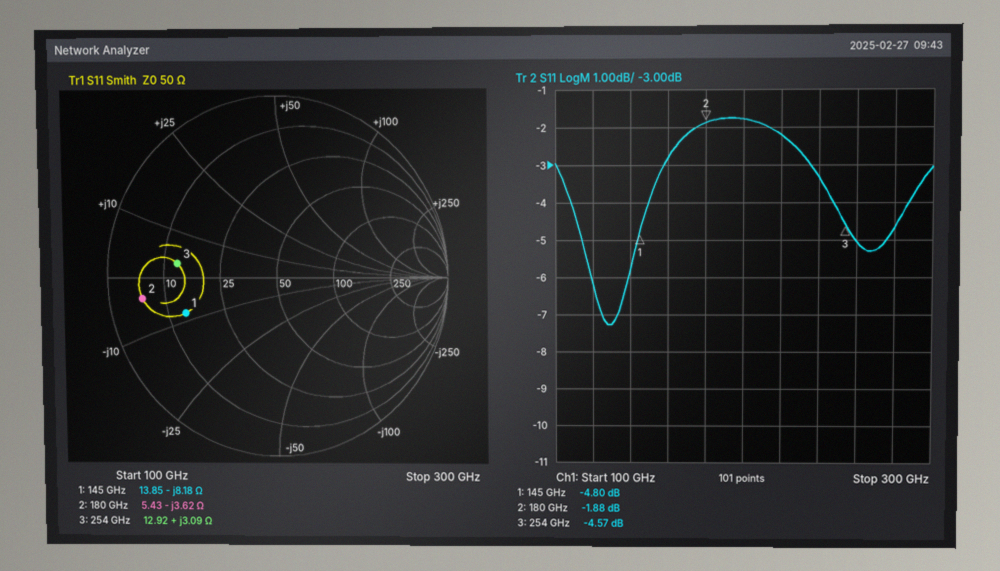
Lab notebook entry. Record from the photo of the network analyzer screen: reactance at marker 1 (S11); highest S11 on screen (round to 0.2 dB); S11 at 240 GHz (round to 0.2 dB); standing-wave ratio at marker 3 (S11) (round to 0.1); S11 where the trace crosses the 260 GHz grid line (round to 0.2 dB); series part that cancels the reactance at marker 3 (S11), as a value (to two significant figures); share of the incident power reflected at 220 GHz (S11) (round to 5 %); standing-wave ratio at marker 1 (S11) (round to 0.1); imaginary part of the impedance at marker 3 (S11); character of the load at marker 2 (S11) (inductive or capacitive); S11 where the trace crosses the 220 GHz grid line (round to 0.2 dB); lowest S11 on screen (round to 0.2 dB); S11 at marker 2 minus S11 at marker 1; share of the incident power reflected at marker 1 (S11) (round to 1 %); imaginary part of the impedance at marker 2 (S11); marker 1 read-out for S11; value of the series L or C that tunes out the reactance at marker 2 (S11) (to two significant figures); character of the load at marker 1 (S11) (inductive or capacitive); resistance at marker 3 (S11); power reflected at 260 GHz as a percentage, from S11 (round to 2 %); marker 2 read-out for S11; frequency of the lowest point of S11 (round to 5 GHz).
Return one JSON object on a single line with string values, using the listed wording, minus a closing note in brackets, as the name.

{"reactance at marker 1": "-8.18 Ω", "highest S11 on screen": "-1.8 dB", "S11 at 240 GHz": "-3.4 dB", "standing-wave ratio at marker 3 (S11)": "3.9", "S11 where the trace crosses the 260 GHz grid line": "-5.0 dB", "series part that cancels the reactance at marker 3 (S11), as a value": "200 fF", "share of the incident power reflected at 220 GHz (S11)": "60 %", "standing-wave ratio at marker 1 (S11)": "3.7", "imaginary part of the impedance at marker 3": "+3.09 Ω", "character of the load at marker 2 (S11)": "capacitive", "S11 where the trace crosses the 220 GHz grid line": "-2.2 dB", "lowest S11 on screen": "-7.2 dB", "S11 at marker 2 minus S11 at marker 1": "2.92 dB", "share of the incident power reflected at marker 1 (S11)": "33 %", "imaginary part of the impedance at marker 2": "-3.62 Ω", "marker 1 read-out for S11": "-4.80 dB", "value of the series L or C that tunes out the reactance at marker 2 (S11)": "3.2 pH", "character of the load at marker 1 (S11)": "capacitive", "resistance at marker 3": "12.92 Ω", "power reflected at 260 GHz as a percentage, from S11": "32 %", "marker 2 read-out for S11": "-1.88 dB", "frequency of the lowest point of S11": "130 GHz"}
